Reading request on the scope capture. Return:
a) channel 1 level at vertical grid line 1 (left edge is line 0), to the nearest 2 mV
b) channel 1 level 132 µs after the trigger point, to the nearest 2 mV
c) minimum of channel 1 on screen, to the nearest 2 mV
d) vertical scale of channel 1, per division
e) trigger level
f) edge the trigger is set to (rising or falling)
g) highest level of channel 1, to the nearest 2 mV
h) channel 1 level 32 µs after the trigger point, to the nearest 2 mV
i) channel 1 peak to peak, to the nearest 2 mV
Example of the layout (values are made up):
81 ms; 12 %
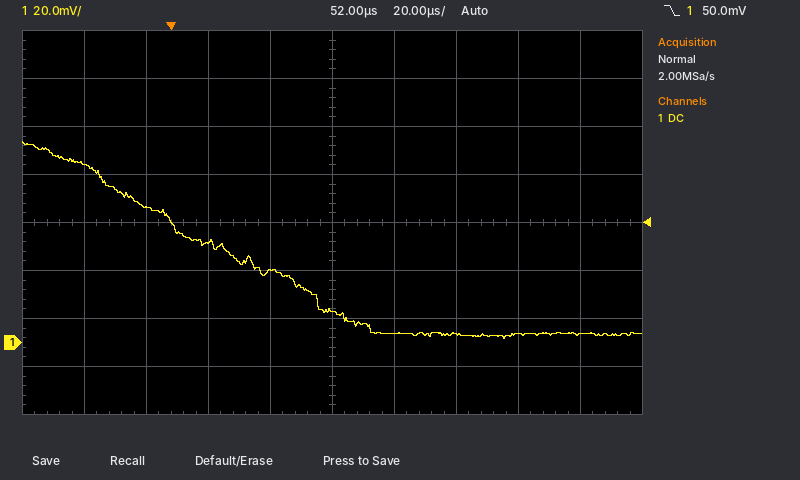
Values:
74 mV; 4 mV; 2 mV; 20 mV; 50.0 mV; falling; 84 mV; 30 mV; 82 mV
